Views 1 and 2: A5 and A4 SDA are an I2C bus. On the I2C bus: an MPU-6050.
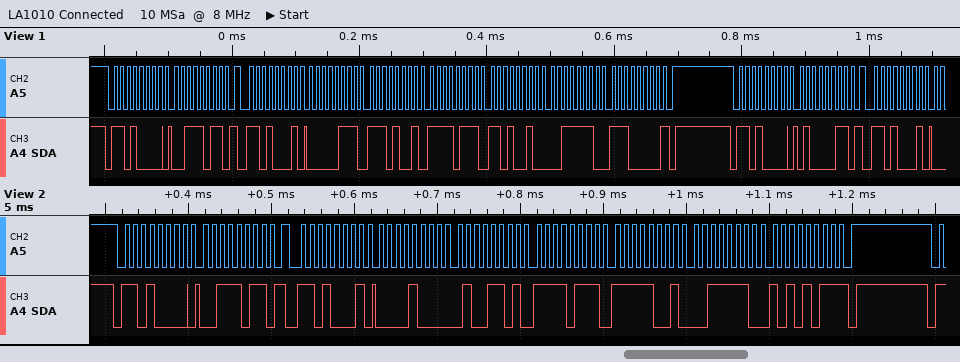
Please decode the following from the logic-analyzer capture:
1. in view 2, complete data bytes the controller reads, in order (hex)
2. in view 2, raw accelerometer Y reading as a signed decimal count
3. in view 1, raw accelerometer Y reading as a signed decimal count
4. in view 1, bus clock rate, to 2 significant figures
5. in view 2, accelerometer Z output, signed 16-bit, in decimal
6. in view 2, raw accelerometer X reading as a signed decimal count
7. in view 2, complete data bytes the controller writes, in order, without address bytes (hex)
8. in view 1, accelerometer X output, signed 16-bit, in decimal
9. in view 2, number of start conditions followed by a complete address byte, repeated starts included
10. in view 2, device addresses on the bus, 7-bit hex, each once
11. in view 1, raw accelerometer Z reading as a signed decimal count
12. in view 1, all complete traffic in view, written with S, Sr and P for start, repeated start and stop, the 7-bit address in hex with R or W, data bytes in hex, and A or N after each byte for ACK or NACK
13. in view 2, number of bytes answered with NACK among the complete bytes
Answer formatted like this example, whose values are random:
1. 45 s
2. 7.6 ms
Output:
1. 08 4D F7 F9 3E AB
2. -2055
3. -2094
4. 100 kHz
5. 16043
6. 2125
7. 3B
8. 2025
9. 2
10. 0x68
11. 16096
12. S 68W A 3B A Sr 68R A 07 A E9 A F7 A D2 A 3E A E0 N P S 68W A 43 A Sr 68R A
13. 1
